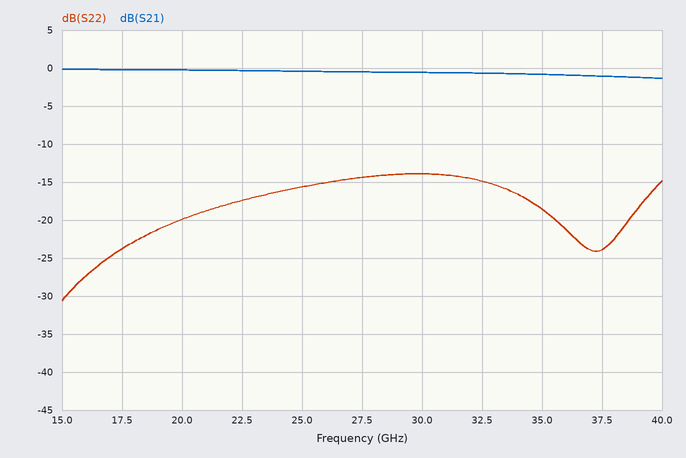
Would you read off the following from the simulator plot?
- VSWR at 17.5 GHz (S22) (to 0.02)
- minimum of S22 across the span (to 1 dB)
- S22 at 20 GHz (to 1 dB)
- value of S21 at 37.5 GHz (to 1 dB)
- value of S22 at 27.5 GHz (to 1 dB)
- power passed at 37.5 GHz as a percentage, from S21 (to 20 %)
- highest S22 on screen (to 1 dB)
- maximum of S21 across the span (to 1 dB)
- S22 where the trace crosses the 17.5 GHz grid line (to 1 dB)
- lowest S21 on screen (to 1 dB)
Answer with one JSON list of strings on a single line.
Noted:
["1.14", "-31 dB", "-20 dB", "-1 dB", "-14 dB", "80 %", "-14 dB", "0 dB", "-24 dB", "-1 dB"]
